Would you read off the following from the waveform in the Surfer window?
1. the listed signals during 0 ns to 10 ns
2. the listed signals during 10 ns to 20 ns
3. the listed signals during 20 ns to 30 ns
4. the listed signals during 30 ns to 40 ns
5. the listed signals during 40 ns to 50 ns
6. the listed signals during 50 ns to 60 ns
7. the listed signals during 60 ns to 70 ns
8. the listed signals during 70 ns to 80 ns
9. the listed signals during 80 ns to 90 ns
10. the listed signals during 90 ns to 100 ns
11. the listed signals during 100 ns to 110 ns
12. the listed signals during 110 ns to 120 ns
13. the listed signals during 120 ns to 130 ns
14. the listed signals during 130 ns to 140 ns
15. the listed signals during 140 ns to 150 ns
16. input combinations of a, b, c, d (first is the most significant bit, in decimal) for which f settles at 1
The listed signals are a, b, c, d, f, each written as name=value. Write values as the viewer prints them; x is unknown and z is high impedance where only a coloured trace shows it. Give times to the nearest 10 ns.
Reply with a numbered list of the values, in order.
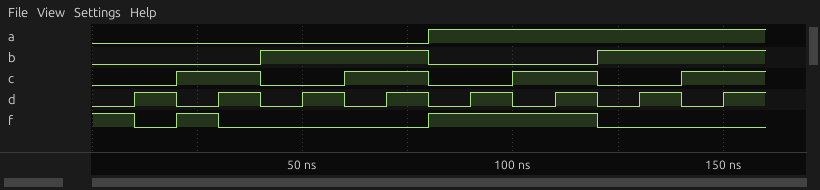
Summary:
1. a=0, b=0, c=0, d=0, f=1
2. a=0, b=0, c=0, d=1, f=0
3. a=0, b=0, c=1, d=0, f=1
4. a=0, b=0, c=1, d=1, f=0
5. a=0, b=1, c=0, d=0, f=0
6. a=0, b=1, c=0, d=1, f=0
7. a=0, b=1, c=1, d=0, f=0
8. a=0, b=1, c=1, d=1, f=0
9. a=1, b=0, c=0, d=0, f=1
10. a=1, b=0, c=0, d=1, f=1
11. a=1, b=0, c=1, d=0, f=1
12. a=1, b=0, c=1, d=1, f=1
13. a=1, b=1, c=0, d=0, f=0
14. a=1, b=1, c=0, d=1, f=0
15. a=1, b=1, c=1, d=0, f=0
16. 0, 2, 8, 9, 10, 11
